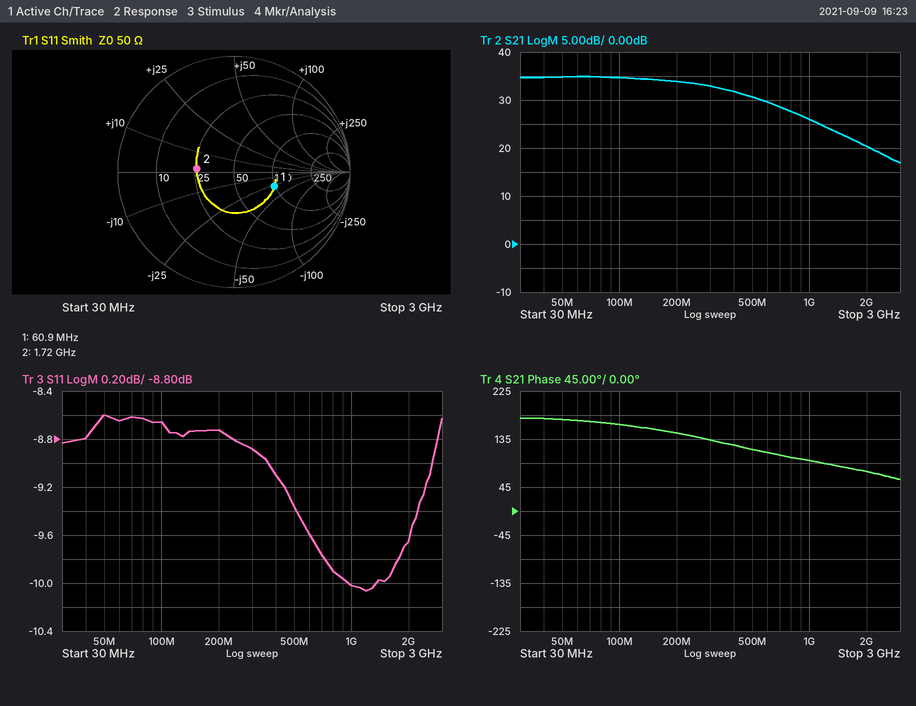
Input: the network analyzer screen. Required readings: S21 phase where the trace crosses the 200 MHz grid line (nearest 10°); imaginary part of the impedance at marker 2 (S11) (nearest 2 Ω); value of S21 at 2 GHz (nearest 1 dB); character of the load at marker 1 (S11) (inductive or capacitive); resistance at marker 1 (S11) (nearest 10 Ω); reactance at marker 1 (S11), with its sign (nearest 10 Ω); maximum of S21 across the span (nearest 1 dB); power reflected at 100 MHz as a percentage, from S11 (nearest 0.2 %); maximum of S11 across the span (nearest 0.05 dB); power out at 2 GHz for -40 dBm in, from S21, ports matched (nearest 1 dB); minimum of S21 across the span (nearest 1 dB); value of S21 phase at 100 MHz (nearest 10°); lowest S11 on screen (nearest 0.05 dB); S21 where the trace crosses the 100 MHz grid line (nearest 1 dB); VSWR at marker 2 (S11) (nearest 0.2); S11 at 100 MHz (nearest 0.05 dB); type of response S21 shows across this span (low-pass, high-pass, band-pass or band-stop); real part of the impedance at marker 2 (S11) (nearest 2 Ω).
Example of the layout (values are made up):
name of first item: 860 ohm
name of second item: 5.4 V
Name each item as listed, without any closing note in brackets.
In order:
S21 phase where the trace crosses the 200 MHz grid line: 150°
imaginary part of the impedance at marker 2 (S11): +2 Ω
value of S21 at 2 GHz: 20 dB
character of the load at marker 1 (S11): capacitive
resistance at marker 1 (S11): 100 Ω
reactance at marker 1 (S11), with its sign: -30 Ω
maximum of S21 across the span: 35 dB
power reflected at 100 MHz as a percentage, from S11: 13.6 %
maximum of S11 across the span: -8.60 dB
power out at 2 GHz for -40 dBm in, from S21, ports matched: -20 dBm
minimum of S21 across the span: 17 dB
value of S21 phase at 100 MHz: 160°
lowest S11 on screen: -10.05 dB
S21 where the trace crosses the 100 MHz grid line: 35 dB
VSWR at marker 2 (S11): 2.0
S11 at 100 MHz: -8.65 dB
type of response S21 shows across this span: low-pass
real part of the impedance at marker 2 (S11): 26 Ω
